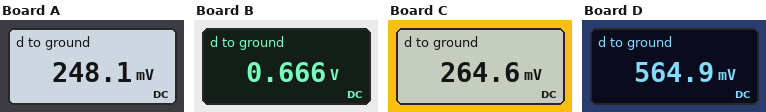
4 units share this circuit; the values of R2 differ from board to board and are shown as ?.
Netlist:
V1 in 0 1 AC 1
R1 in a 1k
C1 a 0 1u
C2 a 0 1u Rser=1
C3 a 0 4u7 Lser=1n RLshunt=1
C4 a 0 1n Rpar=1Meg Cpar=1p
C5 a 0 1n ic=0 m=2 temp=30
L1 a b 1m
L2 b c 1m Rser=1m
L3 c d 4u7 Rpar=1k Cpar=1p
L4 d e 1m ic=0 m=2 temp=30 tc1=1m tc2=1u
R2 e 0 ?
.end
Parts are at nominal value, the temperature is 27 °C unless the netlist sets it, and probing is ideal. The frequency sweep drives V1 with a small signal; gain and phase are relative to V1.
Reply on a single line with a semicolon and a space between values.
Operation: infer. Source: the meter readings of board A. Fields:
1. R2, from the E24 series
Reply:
330 Ω
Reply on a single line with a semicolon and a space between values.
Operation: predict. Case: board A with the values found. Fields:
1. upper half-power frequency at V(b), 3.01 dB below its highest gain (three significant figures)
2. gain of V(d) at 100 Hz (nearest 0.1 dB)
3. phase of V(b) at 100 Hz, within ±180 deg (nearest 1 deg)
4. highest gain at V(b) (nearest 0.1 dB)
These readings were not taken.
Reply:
96.0 Hz; -15.3 dB; -46 deg; -12.1 dB
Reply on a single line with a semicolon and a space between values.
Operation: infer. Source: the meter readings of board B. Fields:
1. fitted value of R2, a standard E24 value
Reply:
2 kΩ
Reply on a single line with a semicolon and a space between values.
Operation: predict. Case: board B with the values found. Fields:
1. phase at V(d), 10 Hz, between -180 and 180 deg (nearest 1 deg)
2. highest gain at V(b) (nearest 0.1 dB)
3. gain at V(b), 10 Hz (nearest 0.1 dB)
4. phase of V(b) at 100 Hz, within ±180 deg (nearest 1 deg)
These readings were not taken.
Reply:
-16 deg; -3.5 dB; -3.9 dB; -70 deg
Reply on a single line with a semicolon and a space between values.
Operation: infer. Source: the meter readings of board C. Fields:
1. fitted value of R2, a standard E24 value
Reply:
360 Ω
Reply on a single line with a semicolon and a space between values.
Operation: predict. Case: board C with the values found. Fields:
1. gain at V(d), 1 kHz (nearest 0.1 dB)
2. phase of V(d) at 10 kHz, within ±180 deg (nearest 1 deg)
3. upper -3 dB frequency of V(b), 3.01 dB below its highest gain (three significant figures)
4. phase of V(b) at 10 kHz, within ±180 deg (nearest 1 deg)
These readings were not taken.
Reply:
-32.5 dB; -108 deg; 90.0 Hz; -98 deg
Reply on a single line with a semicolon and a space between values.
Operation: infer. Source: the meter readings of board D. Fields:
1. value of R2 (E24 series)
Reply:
1.3 kΩ
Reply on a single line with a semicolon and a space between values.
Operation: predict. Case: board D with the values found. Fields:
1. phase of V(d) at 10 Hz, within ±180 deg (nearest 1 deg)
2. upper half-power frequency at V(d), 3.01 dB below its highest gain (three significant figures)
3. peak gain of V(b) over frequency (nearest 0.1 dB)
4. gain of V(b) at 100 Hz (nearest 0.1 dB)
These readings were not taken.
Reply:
-13 deg; 42.0 Hz; -5.0 dB; -13.2 dB
